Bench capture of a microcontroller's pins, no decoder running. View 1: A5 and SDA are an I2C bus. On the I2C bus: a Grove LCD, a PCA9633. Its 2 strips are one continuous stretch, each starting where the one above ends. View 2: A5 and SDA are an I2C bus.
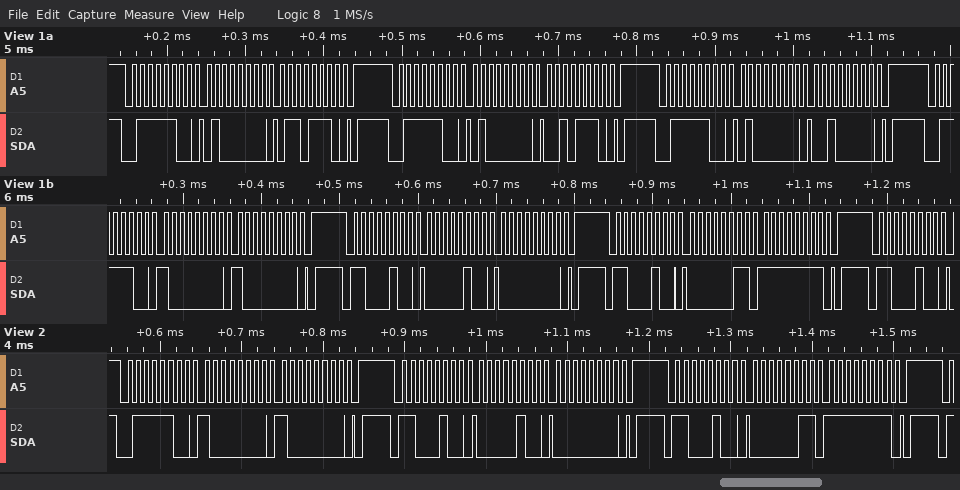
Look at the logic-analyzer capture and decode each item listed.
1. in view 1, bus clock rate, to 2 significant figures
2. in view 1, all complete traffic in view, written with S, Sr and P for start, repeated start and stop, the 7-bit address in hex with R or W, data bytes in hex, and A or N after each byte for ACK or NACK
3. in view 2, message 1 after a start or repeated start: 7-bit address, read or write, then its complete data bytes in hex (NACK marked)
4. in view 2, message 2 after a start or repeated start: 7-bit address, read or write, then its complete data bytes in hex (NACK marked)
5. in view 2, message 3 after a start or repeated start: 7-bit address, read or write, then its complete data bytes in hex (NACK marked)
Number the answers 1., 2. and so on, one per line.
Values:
1. 100 kHz
2. S 3EW A 40 A 6E A P S 3EW A 40 A 2E A P S 3EW A 40 A 20 A P S 3EW A 80 A 80 A P S 62W A 04 A 00 A P S 62W A 03 A FF A P S 62W A
3. 0x3E write: 80 80
4. 0x62 write: 04 00
5. 0x62 write: 03 FF
